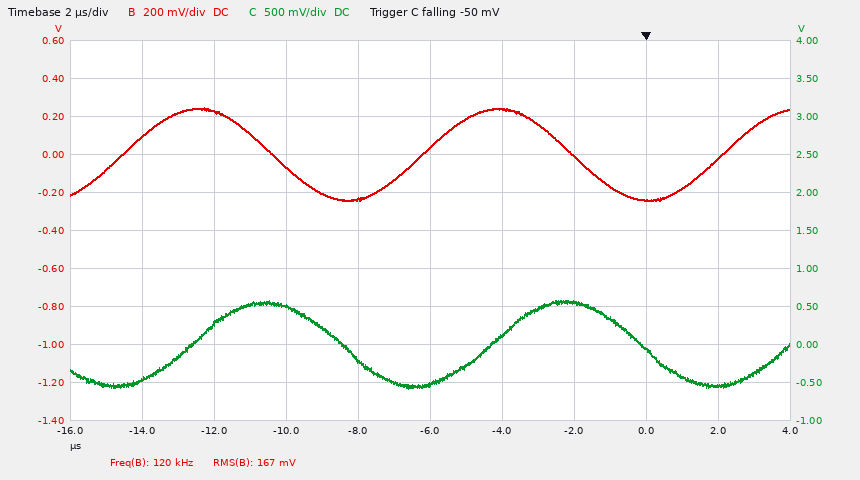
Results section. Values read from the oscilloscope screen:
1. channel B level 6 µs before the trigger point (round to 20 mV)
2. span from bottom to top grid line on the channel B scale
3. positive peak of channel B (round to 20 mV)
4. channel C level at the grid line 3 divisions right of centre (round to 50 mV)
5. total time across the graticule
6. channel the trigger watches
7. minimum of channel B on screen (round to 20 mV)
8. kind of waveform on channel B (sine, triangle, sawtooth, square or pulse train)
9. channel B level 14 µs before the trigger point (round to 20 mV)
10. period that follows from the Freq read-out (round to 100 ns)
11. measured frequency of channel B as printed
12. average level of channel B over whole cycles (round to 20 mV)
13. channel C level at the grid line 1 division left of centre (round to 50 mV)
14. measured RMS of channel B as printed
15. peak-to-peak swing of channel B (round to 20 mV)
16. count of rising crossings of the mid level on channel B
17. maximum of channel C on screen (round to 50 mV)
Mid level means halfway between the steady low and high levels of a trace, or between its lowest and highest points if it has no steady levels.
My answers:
40 mV
2 V
240 mV
-50 mV
20 µs
channel C
-240 mV
sine
100 mV
8.3 µs
120 kHz
0 mV
-200 mV
167 mV
480 mV
3
600 mV
